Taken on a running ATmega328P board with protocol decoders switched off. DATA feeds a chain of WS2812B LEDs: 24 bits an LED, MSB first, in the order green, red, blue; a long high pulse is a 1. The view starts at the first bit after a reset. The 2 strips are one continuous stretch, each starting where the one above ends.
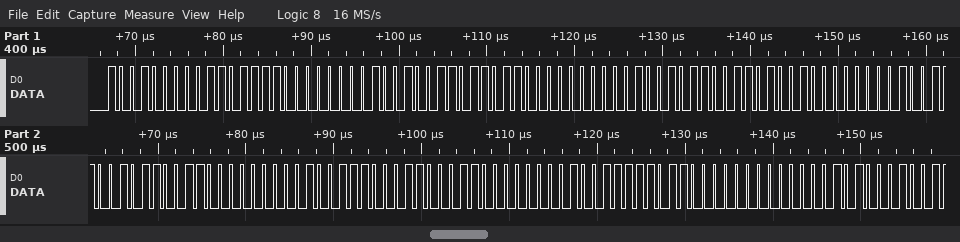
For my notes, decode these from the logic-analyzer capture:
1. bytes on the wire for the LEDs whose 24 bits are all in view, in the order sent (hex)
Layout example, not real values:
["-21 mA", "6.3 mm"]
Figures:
["90 6F 00 93 6C 00 96 69 00 99 66 00 9C 63 00 9F 60 00"]
